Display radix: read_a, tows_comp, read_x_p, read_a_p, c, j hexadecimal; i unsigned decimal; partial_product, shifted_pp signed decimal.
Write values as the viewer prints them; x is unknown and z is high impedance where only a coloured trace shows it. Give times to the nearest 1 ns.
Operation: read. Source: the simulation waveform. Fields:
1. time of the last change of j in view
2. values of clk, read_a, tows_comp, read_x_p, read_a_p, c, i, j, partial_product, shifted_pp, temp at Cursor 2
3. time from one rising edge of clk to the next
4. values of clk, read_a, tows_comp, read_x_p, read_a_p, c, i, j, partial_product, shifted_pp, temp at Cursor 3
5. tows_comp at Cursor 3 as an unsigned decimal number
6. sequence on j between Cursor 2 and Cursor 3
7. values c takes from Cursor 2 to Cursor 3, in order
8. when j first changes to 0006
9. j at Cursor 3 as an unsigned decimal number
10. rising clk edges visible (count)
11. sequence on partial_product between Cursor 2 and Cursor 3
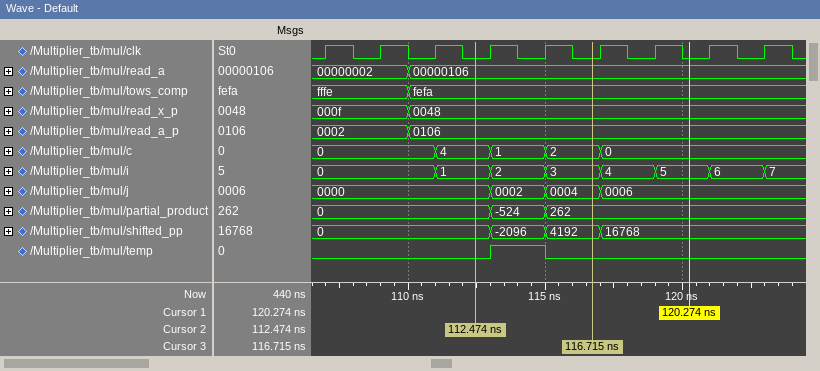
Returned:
117 ns
clk=0, read_a=00000106, tows_comp=fefa, read_x_p=0048, read_a_p=0106, c=4, i=1, j=0000, partial_product=0, shifted_pp=0, temp=0
2 ns
clk=0, read_a=00000106, tows_comp=fefa, read_x_p=0048, read_a_p=0106, c=2, i=3, j=0004, partial_product=262, shifted_pp=4192, temp=0
65274
0000, 0002, 0004
4, 1, 2
117 ns
4
9
0, -524, 262
